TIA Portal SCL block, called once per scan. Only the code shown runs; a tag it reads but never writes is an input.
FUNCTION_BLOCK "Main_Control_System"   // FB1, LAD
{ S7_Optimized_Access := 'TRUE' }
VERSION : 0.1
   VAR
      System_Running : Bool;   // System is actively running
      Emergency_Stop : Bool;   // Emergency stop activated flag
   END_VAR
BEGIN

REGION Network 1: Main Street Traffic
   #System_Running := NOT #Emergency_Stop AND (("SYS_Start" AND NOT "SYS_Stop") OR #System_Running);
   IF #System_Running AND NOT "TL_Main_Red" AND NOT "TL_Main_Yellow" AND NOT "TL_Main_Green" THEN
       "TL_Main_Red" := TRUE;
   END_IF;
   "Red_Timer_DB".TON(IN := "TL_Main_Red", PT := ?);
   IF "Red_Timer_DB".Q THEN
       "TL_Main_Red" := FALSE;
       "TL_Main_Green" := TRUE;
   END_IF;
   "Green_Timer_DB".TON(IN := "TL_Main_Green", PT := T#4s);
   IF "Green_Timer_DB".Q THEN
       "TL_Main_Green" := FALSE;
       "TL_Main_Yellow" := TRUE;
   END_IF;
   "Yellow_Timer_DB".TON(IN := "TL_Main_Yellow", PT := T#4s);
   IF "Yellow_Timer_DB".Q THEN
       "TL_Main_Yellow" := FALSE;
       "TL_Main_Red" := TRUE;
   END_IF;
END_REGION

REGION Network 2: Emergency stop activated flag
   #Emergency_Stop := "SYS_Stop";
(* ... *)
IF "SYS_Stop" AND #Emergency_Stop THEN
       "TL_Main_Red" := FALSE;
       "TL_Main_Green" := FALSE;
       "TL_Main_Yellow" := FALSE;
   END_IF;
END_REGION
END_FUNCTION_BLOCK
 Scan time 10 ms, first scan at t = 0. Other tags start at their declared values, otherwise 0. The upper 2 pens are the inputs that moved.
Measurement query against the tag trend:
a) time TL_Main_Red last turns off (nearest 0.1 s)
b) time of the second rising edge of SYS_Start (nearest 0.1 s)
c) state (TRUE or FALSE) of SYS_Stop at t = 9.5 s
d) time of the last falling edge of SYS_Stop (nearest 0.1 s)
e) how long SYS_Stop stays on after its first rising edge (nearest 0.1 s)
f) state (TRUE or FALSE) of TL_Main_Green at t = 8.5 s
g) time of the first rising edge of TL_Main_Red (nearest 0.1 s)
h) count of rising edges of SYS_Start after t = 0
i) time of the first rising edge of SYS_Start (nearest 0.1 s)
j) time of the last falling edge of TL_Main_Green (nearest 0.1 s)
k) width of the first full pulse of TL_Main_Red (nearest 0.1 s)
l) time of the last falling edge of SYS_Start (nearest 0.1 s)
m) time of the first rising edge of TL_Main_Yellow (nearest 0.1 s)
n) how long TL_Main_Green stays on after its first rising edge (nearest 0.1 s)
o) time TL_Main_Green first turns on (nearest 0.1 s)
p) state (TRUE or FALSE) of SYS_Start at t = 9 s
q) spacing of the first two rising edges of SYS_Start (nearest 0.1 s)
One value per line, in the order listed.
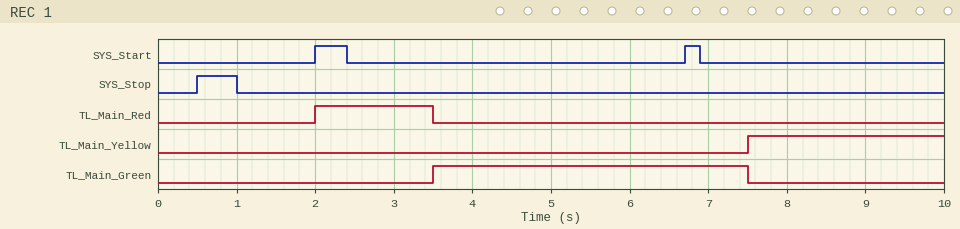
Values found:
3.5 s
6.7 s
FALSE
1.0 s
0.5 s
FALSE
2.0 s
2
2.0 s
7.5 s
1.5 s
6.9 s
7.5 s
4.0 s
3.5 s
FALSE
4.7 s
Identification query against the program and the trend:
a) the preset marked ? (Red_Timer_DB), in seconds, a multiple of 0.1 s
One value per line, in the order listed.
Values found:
1.5 s
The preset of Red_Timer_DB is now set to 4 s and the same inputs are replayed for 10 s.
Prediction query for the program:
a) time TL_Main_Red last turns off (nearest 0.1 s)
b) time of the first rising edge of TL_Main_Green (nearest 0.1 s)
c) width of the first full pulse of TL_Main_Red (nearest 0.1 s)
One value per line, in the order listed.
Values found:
6.0 s
6.0 s
4.0 s
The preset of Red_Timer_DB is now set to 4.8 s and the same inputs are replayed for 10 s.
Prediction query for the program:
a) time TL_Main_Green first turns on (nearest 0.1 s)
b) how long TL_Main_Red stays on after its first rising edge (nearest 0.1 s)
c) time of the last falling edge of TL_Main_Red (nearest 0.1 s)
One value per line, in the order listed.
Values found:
6.8 s
4.8 s
6.8 s
